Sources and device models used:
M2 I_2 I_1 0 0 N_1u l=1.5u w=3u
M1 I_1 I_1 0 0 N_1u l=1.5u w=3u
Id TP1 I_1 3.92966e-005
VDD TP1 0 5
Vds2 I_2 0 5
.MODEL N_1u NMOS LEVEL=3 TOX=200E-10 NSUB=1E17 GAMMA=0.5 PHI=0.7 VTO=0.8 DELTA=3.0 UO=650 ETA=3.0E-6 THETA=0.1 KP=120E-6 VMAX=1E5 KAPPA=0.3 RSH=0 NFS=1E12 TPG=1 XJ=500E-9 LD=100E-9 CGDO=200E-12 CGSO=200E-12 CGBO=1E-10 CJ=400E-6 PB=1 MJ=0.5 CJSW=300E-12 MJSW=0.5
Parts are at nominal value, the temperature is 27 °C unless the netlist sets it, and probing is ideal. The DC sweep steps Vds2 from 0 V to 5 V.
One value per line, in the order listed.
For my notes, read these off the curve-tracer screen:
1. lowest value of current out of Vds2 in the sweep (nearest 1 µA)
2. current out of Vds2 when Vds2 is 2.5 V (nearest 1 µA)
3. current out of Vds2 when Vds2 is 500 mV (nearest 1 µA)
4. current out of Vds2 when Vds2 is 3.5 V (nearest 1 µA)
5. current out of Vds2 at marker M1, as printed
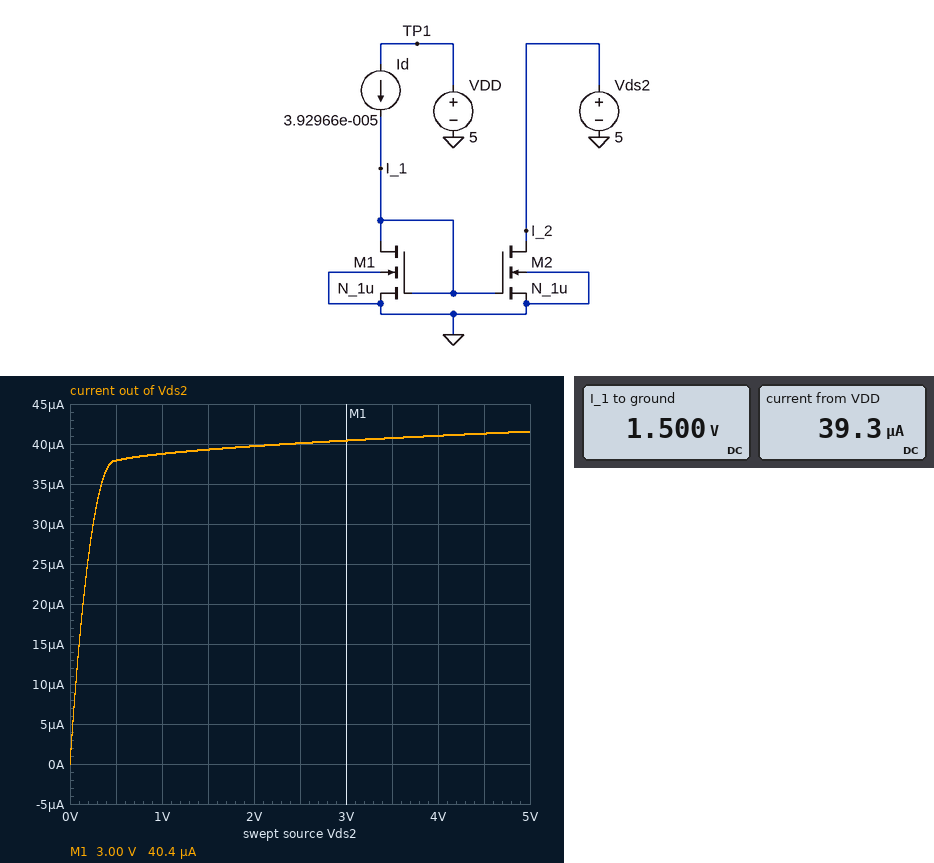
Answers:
0 A
40 µA
38 µA
41 µA
40.4 µA
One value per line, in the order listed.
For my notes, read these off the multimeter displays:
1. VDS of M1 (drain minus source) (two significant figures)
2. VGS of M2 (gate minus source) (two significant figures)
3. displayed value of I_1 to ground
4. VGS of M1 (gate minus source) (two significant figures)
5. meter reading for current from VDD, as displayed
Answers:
1.5 V
1.5 V
1.500 V
1.5 V
39.3 µA
